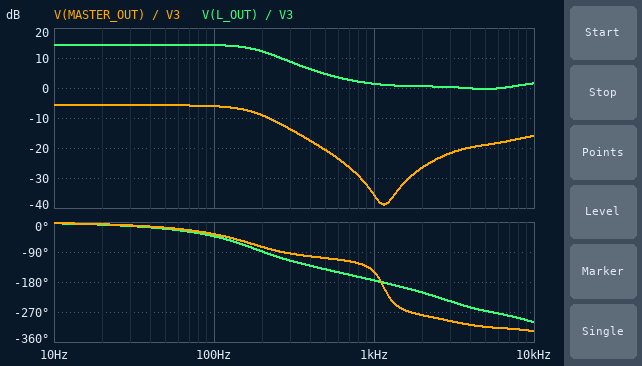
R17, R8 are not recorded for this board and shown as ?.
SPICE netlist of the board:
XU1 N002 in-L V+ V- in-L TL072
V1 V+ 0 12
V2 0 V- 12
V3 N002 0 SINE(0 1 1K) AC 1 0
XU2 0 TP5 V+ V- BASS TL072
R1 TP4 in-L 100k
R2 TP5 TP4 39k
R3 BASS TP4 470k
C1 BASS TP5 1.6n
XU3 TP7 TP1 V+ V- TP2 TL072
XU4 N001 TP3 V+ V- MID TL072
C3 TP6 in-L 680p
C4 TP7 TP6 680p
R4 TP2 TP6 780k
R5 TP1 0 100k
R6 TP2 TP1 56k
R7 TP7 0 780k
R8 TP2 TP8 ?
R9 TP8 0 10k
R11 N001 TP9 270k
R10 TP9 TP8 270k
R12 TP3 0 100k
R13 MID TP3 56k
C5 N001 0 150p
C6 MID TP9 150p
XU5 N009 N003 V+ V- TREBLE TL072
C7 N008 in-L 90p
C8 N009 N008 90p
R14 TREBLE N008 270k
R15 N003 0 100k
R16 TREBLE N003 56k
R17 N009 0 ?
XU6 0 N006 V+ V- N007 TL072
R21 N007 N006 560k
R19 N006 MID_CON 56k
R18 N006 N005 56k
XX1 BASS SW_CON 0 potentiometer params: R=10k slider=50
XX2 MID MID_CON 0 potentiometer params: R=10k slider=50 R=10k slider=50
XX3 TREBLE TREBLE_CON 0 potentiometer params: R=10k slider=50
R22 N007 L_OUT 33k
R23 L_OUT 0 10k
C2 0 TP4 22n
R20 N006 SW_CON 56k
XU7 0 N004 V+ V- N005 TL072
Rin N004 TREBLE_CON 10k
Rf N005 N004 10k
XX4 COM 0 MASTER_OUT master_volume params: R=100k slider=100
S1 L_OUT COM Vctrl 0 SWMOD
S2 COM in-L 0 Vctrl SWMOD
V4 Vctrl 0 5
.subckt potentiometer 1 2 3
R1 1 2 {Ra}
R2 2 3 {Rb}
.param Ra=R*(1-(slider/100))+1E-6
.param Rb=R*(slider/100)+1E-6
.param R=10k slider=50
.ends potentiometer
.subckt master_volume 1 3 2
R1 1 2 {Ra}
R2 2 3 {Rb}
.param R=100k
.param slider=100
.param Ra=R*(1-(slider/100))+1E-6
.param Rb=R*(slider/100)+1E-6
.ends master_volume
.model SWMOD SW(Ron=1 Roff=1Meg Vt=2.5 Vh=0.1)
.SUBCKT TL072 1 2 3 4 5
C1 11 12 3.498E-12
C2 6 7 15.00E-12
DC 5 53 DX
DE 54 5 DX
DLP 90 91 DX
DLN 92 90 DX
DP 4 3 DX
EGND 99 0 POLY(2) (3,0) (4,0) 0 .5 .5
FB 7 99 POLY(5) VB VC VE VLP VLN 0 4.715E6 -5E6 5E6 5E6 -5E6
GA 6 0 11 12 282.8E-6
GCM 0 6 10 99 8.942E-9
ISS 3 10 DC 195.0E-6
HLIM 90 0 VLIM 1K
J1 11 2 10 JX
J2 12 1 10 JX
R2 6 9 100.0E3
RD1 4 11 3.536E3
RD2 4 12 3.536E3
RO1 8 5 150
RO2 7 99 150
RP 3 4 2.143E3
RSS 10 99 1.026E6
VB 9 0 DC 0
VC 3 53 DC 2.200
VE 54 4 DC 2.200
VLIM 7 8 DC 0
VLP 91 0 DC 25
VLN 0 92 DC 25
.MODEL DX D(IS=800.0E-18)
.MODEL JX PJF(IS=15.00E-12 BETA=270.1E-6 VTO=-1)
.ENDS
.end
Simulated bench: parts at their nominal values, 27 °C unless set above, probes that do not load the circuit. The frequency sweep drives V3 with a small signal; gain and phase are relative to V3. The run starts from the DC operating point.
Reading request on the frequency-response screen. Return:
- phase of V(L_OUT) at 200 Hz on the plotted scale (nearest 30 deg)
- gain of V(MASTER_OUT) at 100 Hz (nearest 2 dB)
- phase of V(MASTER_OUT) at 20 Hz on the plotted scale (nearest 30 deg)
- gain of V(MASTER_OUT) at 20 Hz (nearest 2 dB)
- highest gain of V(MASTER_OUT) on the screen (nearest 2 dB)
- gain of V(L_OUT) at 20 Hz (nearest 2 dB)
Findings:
-90 deg
-6 dB
0 deg
-6 dB
-6 dB
14 dB
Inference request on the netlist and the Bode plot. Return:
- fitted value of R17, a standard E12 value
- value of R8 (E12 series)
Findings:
220 kΩ
18 kΩ
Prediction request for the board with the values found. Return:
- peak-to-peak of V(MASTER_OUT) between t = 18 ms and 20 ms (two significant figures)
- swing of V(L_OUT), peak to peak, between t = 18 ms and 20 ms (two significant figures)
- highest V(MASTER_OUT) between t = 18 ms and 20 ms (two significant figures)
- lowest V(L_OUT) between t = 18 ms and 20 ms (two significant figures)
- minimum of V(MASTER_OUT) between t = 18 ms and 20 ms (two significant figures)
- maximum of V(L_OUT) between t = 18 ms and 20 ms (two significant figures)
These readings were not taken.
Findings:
2.2 V
2.2 V
1.1 V
-1.1 V
-1.1 V
1.1 V
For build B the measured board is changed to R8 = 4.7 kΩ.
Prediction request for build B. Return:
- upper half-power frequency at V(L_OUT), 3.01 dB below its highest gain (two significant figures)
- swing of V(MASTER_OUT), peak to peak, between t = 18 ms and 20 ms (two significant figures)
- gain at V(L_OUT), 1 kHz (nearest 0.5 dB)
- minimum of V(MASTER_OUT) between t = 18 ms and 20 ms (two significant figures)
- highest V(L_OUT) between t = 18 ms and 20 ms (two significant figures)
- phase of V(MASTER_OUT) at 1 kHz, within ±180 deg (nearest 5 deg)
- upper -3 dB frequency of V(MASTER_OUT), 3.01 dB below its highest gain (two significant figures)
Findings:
250 Hz
3.8 V
6.0 dB
-1.9 V
1.9 V
-170 deg
210 Hz
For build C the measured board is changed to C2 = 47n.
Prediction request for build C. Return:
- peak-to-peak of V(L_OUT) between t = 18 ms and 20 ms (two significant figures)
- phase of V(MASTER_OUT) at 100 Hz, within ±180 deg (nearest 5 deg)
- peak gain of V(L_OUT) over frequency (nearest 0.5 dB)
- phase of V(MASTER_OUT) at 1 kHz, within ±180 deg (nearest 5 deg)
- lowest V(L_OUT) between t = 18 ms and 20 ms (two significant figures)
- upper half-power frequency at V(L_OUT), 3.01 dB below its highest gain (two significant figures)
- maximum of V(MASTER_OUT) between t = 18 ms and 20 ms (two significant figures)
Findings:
2.0 V
-50 deg
16.0 dB
-140 deg
-990 mV
160 Hz
990 mV
